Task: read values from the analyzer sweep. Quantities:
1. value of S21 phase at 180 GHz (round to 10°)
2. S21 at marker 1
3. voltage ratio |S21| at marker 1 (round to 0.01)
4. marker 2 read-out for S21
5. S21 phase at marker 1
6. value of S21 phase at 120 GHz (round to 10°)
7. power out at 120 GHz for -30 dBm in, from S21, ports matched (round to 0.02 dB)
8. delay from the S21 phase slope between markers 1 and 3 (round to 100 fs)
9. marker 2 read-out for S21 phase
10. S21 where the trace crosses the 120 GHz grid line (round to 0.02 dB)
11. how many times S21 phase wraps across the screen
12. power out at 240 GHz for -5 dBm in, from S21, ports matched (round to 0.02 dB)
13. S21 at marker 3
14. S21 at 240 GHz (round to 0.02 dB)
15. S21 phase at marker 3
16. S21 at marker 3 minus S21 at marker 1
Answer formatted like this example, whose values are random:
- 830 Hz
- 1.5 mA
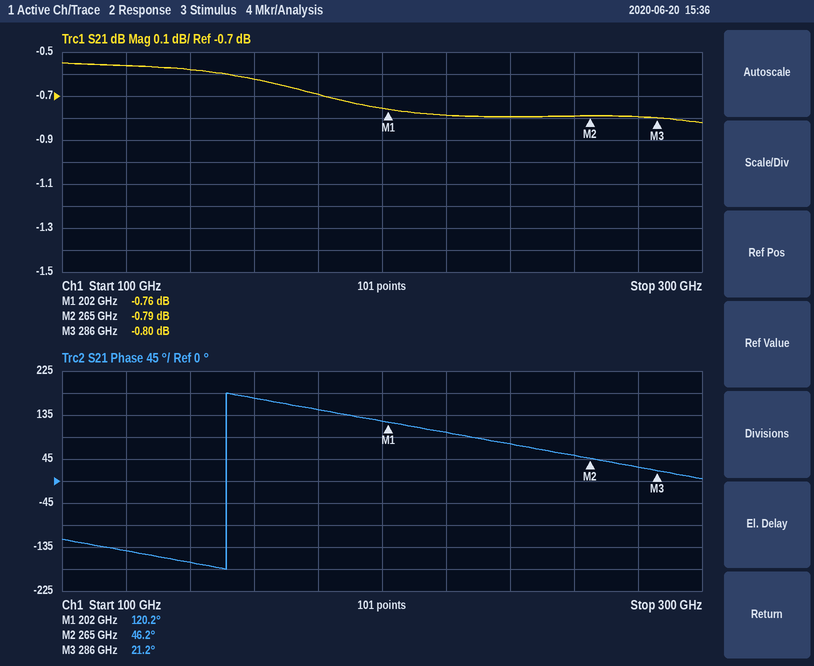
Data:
- 150°
- -0.76 dB
- 0.92
- -0.79 dB
- 120.2°
- -140°
- -30.56 dBm
- 3.3 ps
- 46.2°
- -0.56 dB
- 1
- -5.80 dBm
- -0.80 dB
- -0.80 dB
- 21.2°
- -0.04 dB
